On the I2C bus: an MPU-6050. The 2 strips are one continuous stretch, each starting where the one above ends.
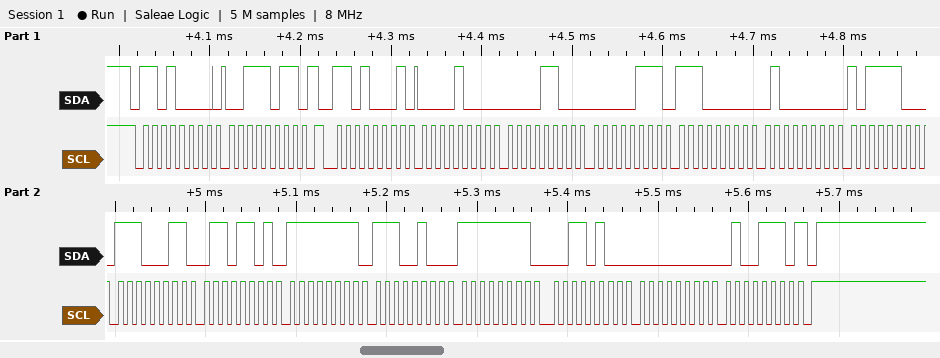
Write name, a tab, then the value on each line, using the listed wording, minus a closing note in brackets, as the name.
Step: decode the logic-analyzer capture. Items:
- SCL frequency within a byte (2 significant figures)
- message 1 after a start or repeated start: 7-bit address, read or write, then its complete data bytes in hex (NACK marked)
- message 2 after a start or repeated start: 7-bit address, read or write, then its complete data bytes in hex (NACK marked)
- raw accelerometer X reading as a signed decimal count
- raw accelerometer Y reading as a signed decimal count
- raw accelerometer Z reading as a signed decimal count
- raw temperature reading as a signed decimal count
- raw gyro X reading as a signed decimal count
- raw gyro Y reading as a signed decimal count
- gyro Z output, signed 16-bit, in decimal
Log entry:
SCL frequency within a byte	100 kHz
message 1 after a start or repeated start: 7-bit address, read or write, then its complete data bytes in hex	0x68 write: 3B
message 2 after a start or repeated start: 7-bit address, read or write, then its complete data bytes in hex	0x68 read: 08 0C 07 E0 40 BC E3 6D FF E4 FF 34 00 4E NACK
raw accelerometer X reading as a signed decimal count	2060
raw accelerometer Y reading as a signed decimal count	2016
raw accelerometer Z reading as a signed decimal count	16572
raw temperature reading as a signed decimal count	-7315
raw gyro X reading as a signed decimal count	-28
raw gyro Y reading as a signed decimal count	-204
gyro Z output, signed 16-bit, in decimal	78
